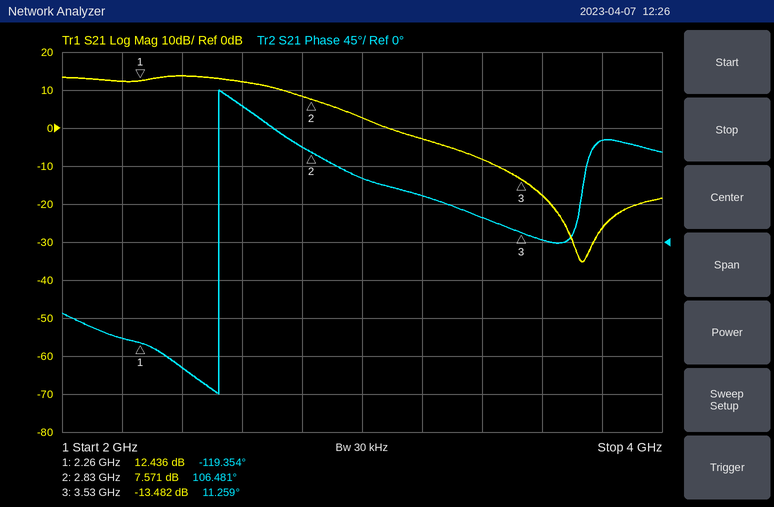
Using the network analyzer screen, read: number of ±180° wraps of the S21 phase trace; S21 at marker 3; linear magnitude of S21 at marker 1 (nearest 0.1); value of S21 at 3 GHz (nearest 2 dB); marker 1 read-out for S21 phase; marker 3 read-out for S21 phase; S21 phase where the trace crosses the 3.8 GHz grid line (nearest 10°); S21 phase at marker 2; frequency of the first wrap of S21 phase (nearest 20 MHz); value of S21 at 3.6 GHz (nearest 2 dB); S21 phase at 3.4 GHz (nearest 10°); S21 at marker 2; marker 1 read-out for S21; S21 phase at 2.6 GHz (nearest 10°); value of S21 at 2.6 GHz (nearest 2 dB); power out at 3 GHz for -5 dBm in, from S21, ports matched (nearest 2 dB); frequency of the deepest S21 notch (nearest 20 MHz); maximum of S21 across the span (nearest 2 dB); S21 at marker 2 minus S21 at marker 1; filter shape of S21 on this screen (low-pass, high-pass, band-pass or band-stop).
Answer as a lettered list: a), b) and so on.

a) 1
b) -13.482 dB
c) 4.2
d) 2 dB
e) -119.354°
f) 11.259°
g) 120°
h) 106.481°
i) 2.52 GHz
j) -18 dB
k) 30°
l) 7.571 dB
m) 12.436 dB
n) 160°
o) 12 dB
p) -2 dBm
q) 3.74 GHz
r) 14 dB
s) -4.865 dB
t) low-pass
